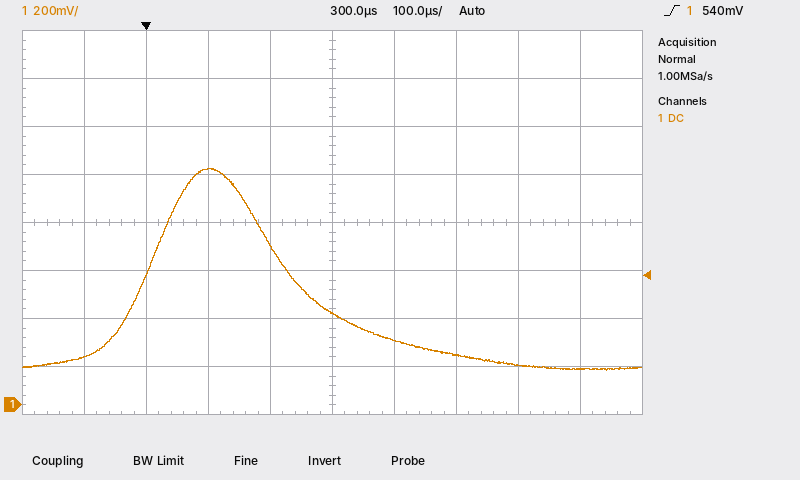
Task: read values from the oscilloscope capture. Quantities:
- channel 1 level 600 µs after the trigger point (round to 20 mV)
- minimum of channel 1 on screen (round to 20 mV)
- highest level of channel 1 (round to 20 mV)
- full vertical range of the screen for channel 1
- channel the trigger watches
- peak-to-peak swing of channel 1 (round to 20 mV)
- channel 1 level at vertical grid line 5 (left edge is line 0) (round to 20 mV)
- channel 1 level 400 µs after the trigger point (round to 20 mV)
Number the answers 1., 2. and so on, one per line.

1. 160 mV
2. 140 mV
3. 980 mV
4. 1.6 V
5. channel 1
6. 840 mV
7. 380 mV
8. 260 mV
